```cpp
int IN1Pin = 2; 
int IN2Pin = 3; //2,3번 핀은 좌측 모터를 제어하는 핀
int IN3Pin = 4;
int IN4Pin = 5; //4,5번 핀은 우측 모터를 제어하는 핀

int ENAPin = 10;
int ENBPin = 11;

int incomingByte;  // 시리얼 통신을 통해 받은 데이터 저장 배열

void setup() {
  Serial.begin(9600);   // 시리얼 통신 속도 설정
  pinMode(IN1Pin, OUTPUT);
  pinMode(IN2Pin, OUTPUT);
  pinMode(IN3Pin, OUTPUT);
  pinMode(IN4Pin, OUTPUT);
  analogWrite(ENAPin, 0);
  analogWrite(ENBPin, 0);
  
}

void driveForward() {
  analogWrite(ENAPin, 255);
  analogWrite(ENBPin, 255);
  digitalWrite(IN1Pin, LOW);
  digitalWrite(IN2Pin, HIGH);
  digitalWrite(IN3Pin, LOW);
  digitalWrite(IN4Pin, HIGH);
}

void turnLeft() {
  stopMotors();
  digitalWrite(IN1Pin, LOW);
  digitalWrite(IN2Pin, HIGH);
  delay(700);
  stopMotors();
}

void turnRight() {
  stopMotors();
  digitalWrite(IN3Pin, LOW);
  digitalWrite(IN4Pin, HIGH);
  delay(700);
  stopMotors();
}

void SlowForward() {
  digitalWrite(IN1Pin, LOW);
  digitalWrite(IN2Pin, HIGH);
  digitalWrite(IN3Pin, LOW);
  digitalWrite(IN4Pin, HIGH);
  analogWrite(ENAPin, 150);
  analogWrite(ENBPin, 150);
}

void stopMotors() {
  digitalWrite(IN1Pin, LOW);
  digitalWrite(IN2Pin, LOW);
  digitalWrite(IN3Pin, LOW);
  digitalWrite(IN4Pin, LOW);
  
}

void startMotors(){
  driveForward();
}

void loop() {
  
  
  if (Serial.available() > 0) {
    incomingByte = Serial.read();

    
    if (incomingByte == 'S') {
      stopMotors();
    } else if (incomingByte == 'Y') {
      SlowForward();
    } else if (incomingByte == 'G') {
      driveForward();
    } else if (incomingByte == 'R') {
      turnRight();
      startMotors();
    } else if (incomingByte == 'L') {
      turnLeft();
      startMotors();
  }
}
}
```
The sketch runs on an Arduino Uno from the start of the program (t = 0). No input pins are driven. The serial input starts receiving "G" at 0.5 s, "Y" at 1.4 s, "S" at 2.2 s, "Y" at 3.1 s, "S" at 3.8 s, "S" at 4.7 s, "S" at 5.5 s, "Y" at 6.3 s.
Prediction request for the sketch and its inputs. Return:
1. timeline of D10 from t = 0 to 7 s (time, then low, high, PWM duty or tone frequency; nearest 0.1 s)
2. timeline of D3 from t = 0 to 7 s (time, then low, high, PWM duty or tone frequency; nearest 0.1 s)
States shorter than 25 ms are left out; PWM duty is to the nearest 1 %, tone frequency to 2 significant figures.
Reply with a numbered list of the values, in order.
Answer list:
1. 0 s low; 0.5 s high; 1.4 s PWM 59 %
2. 0 s low; 0.5 s high; 2.2 s low; 3.1 s high; 3.8 s low; 6.3 s high
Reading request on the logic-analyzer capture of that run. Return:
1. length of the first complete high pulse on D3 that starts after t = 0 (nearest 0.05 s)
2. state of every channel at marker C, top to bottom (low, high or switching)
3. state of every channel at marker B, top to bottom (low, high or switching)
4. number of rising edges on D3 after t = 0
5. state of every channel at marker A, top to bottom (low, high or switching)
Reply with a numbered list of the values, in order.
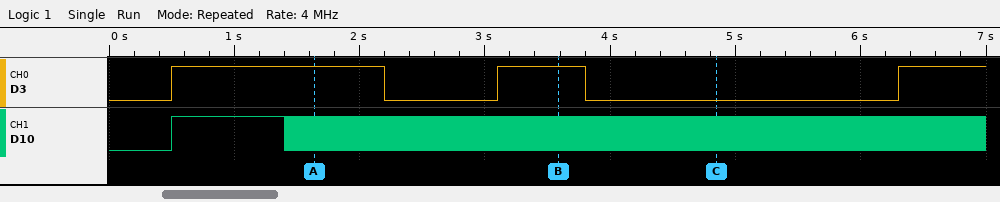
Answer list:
1. 1.70 s
2. D3 low, D10 switching
3. D3 high, D10 switching
4. 3
5. D3 high, D10 switching
